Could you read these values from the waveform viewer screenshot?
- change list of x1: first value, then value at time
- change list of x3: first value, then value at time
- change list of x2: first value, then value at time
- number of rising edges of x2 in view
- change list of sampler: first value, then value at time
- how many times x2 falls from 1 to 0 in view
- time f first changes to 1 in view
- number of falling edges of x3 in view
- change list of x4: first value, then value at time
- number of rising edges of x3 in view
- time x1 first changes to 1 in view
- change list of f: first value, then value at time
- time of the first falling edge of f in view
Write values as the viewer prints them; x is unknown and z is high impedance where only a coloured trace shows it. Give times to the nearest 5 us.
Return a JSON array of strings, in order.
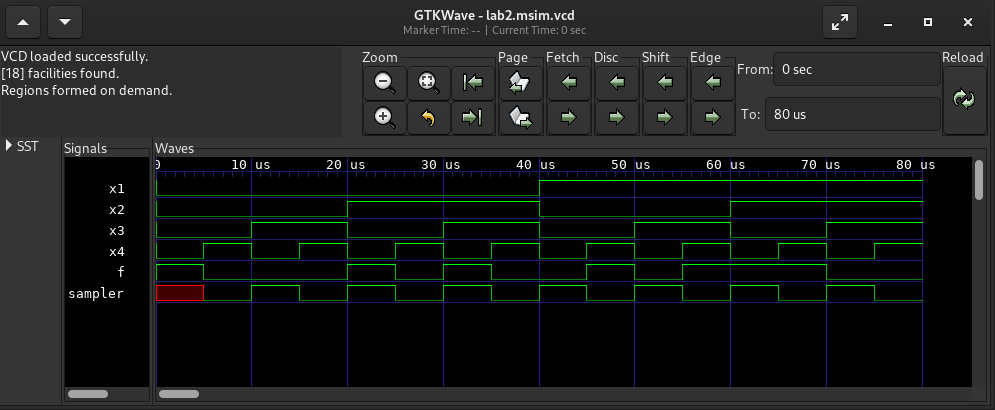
["0, 1 at 40 us", "0, 1 at 10 us, 0 at 20 us, 1 at 30 us, 0 at 40 us, 1 at 50 us, 0 at 60 us, 1 at 70 us", "0, 1 at 20 us, 0 at 40 us, 1 at 60 us", "2", "x, 0 at 5 us, 1 at 10 us, 0 at 15 us, 1 at 20 us, 0 at 25 us, 1 at 30 us, 0 at 35 us, 1 at 40 us, 0 at 45 us, 1 at 50 us, 0 at 55 us, 1 at 60 us, 0 at 65 us, 1 at 70 us, 0 at 75 us", "1", "20 us", "3", "0, 1 at 5 us, 0 at 10 us, 1 at 15 us, 0 at 20 us, 1 at 25 us, 0 at 30 us, 1 at 35 us, 0 at 40 us, 1 at 45 us, 0 at 50 us, 1 at 55 us, 0 at 60 us, 1 at 65 us, 0 at 70 us, 1 at 75 us", "4", "40 us", "1, 0 at 5 us, 1 at 20 us, 0 at 25 us, 1 at 30 us, 0 at 35 us, 1 at 45 us, 0 at 50 us, 1 at 55 us, 0 at 70 us", "5 us"]
